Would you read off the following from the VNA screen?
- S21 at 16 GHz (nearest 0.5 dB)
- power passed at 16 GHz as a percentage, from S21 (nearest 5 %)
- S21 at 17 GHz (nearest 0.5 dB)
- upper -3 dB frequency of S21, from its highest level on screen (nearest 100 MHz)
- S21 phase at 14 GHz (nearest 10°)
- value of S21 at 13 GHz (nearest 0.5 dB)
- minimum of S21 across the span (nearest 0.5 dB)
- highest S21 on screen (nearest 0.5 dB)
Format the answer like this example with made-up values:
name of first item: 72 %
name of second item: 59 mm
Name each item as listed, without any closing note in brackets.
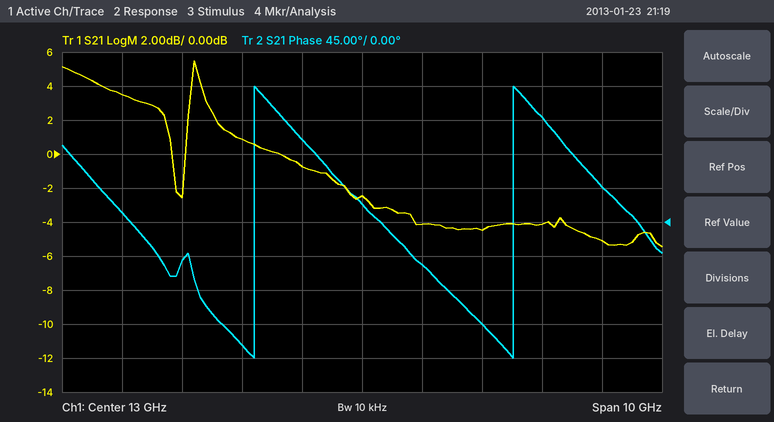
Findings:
S21 at 16 GHz: -4.0 dB
power passed at 16 GHz as a percentage, from S21: 40 %
S21 at 17 GHz: -5.0 dB
upper -3 dB frequency of S21, from its highest level on screen: 10.5 GHz
S21 phase at 14 GHz: -60°
value of S21 at 13 GHz: -2.5 dB
minimum of S21 across the span: -5.5 dB
highest S21 on screen: 5.5 dB
